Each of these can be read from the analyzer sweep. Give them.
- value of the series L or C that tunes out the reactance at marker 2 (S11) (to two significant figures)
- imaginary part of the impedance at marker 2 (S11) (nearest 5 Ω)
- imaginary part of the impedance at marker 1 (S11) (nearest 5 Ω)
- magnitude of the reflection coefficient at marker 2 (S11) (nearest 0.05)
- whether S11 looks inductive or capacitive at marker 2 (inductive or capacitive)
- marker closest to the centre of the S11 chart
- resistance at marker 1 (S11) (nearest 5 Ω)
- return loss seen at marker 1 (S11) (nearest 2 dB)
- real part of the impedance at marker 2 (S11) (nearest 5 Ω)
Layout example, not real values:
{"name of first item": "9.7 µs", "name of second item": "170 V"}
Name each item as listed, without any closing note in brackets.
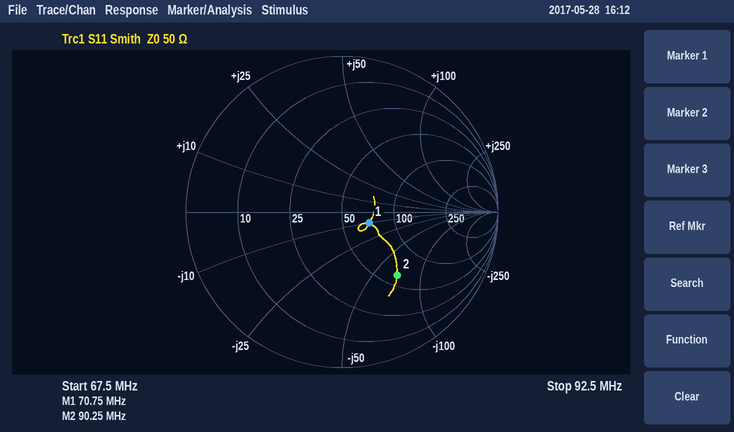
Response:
{"value of the series L or C that tunes out the reactance at marker 2 (S11)": "120 nH", "imaginary part of the impedance at marker 2 (S11)": "-70 Ω", "imaginary part of the impedance at marker 1 (S11)": "-10 Ω", "magnitude of the reflection coefficient at marker 2 (S11)": "0.55", "whether S11 looks inductive or capacitive at marker 2": "capacitive", "marker closest to the centre of the S11 chart": "marker 1", "resistance at marker 1 (S11)": "70 Ω", "return loss seen at marker 1 (S11)": "14 dB", "real part of the impedance at marker 2 (S11)": "60 Ω"}
